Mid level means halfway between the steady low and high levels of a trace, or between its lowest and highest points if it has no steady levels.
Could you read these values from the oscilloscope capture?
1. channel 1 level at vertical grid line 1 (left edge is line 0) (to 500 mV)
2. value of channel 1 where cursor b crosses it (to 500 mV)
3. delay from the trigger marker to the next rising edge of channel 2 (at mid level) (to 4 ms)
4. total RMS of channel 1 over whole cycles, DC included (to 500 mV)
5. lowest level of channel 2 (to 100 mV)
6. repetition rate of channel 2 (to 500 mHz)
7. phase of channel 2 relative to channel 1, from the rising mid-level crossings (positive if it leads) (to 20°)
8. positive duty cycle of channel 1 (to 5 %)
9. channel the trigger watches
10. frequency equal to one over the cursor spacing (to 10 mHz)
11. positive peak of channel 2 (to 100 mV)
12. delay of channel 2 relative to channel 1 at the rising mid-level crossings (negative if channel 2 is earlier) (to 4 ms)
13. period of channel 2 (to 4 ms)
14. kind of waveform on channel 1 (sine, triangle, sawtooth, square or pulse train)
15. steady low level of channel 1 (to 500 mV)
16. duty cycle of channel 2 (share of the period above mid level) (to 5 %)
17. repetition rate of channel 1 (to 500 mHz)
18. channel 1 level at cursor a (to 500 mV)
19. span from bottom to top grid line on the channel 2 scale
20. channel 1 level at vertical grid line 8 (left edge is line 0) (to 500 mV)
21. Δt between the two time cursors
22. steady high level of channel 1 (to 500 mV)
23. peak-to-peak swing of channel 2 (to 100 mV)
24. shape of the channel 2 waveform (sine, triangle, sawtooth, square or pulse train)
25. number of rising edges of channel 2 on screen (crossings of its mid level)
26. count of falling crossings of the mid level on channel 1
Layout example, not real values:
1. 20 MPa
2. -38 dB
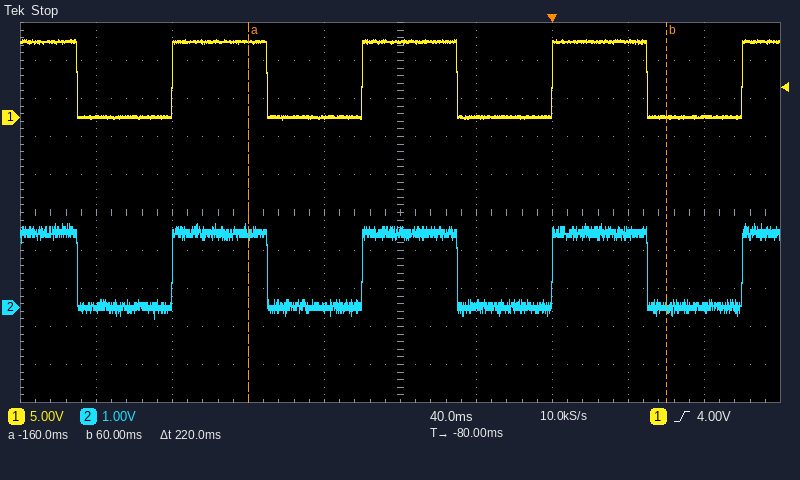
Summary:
1. 0.0 V
2. 0.0 V
3. 100 ms
4. 7.0 V
5. -300 mV
6. 10.0 Hz
7. 0°
8. 50 %
9. channel 1
10. 4.55 Hz
11. 2.2 V
12. 0 ms
13. 100 ms
14. square
15. 0.0 V
16. 50 %
17. 10.0 Hz
18. 10.0 V
19. 10 V
20. 10.0 V
21. 220 ms
22. 10.0 V
23. 2.5 V
24. square
25. 4
26. 4
